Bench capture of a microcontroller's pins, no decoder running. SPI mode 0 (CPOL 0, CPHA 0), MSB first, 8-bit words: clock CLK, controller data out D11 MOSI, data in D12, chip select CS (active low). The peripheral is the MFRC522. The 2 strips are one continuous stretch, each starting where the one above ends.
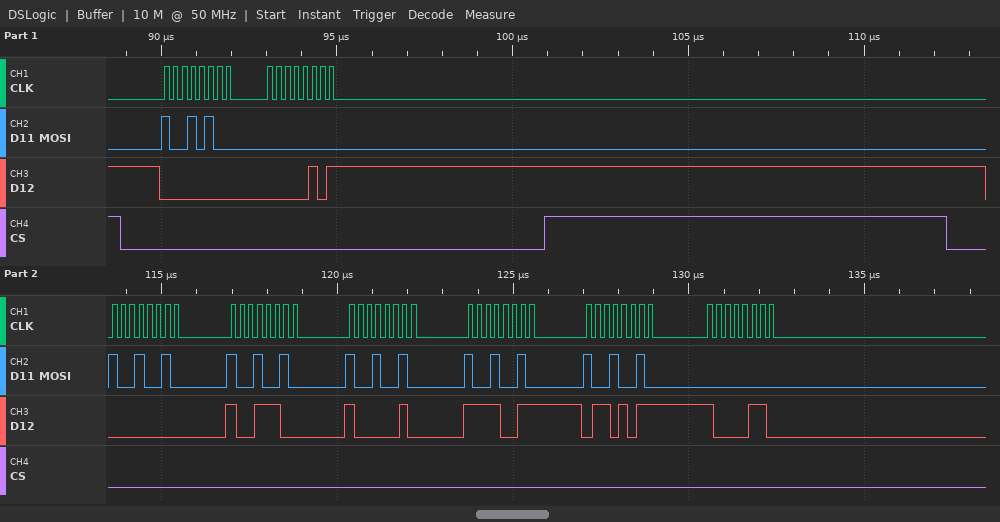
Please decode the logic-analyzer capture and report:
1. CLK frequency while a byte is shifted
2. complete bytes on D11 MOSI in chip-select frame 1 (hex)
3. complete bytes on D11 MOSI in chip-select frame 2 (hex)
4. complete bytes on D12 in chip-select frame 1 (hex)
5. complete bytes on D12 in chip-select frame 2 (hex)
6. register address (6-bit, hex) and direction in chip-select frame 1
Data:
4 MHz
0x94 0x00
0x92 0x92 0x92 0x92 0x92 0x00
0x00 0x05
0x00 0x9C 0x82 0xF3 0x6B 0x86
0x0A read
